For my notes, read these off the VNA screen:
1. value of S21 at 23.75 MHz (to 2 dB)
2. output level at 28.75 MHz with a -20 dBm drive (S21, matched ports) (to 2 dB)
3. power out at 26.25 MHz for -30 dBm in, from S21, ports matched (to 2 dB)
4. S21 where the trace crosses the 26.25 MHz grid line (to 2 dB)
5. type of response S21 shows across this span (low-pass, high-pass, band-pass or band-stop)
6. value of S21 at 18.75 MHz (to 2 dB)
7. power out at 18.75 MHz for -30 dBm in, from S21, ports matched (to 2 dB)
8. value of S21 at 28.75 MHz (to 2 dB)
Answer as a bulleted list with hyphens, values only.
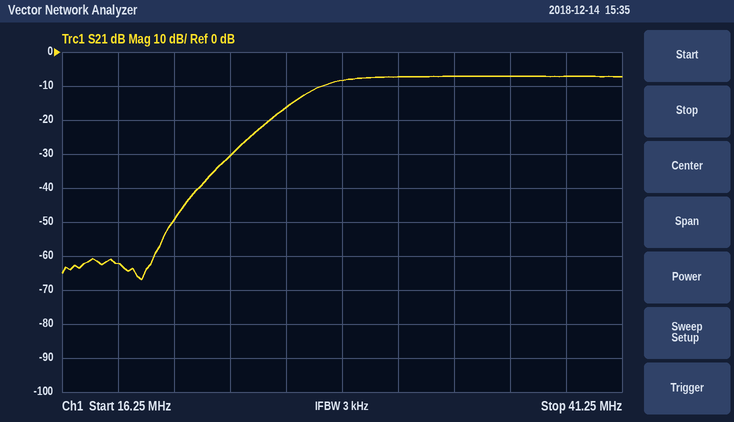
- -30 dB
- -28 dBm
- -46 dBm
- -16 dB
- high-pass
- -62 dB
- -92 dBm
- -8 dB
